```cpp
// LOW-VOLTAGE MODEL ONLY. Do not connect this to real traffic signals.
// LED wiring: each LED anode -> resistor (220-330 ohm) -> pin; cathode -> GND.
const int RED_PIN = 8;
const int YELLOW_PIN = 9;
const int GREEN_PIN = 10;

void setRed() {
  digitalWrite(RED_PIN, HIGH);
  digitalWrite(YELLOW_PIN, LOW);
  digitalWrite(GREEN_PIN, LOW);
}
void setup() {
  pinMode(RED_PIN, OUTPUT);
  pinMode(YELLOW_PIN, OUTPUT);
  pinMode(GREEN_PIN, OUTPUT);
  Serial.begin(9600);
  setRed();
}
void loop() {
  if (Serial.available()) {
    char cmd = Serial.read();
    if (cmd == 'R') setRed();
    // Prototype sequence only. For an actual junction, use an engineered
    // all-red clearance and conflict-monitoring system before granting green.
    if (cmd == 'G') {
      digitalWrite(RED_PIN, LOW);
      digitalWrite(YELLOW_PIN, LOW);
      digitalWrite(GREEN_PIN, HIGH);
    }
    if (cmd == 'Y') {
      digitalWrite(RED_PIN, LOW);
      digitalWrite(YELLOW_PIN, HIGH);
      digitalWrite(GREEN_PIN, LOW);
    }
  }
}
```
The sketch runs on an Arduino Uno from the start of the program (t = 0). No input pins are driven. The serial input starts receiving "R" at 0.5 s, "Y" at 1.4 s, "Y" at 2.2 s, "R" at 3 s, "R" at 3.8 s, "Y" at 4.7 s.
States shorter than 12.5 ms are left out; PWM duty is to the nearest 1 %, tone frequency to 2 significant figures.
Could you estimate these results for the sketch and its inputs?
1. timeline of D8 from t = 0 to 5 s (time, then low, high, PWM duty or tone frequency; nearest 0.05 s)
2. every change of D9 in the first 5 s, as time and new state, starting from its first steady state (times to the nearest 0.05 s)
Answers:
0 s high; 1.4 s low; 3 s high; 4.7 s low
0 s low; 1.4 s high; 3 s low; 4.7 s high
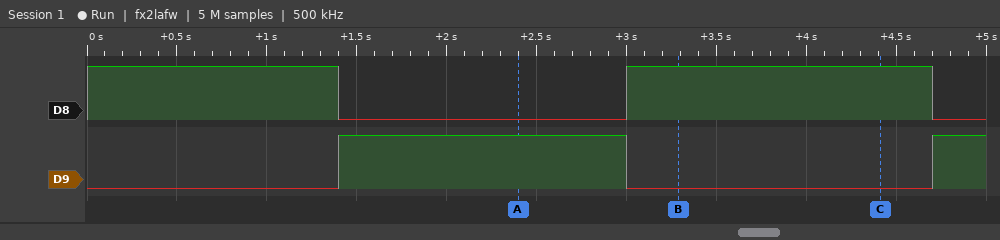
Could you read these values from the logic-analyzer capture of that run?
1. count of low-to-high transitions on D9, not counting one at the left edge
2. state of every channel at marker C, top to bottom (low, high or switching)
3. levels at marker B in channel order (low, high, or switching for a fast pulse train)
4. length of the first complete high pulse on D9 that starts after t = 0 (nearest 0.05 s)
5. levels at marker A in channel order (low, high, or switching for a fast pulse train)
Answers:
2
D8 high, D9 low
D8 high, D9 low
1.60 s
D8 low, D9 high
